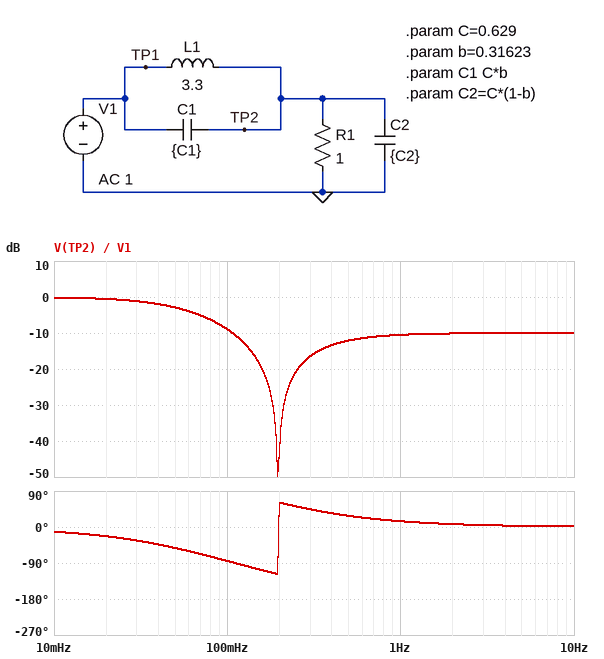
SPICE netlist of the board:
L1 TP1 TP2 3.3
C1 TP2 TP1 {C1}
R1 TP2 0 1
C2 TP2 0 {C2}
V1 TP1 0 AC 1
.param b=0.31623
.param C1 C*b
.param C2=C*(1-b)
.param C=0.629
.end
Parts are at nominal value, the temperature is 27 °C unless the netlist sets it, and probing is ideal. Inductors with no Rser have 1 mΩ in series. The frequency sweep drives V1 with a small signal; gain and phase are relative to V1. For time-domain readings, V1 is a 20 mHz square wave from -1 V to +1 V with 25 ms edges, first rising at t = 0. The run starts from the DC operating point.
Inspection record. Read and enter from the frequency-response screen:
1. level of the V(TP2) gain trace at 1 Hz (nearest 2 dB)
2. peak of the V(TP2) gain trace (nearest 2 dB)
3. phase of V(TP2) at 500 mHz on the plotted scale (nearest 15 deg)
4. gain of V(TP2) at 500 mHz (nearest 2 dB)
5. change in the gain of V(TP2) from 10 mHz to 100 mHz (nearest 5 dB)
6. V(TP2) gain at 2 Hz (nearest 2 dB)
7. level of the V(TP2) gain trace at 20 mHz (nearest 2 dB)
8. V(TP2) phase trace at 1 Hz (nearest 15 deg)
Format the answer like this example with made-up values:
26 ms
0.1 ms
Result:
-10 dB
0 dB
30 deg
-12 dB
-10 dB
-10 dB
0 dB
15 deg
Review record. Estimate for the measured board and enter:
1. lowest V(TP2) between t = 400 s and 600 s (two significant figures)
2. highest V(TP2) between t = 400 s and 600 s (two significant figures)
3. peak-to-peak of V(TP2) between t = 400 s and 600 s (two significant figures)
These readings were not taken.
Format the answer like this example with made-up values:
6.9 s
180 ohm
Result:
-1.0 V
1.0 V
2.0 V
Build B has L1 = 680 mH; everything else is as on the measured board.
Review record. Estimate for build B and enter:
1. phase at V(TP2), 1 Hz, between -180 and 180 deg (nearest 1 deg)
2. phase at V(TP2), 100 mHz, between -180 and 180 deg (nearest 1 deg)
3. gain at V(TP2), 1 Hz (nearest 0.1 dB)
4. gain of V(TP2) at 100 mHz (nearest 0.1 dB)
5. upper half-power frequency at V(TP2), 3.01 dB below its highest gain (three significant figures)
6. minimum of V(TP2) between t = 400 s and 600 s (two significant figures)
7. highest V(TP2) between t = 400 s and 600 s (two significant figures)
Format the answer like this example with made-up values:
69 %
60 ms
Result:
15 deg
-27 deg
-11.6 dB
0.1 dB
232 mHz
-1.2 V
1.2 V
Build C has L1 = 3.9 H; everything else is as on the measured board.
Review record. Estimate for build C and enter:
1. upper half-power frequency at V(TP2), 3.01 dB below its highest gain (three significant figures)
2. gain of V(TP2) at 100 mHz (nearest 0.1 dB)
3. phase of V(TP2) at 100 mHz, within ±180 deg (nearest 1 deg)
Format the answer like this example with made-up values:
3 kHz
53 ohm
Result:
42.9 mHz
-11.0 dB
-89 deg
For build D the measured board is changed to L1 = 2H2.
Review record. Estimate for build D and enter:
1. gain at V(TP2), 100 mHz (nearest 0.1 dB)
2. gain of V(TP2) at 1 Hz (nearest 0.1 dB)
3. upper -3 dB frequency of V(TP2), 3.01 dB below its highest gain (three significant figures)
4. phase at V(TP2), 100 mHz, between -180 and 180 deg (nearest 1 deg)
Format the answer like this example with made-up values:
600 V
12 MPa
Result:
-4.9 dB
-10.6 dB
77.8 mHz
-72 deg
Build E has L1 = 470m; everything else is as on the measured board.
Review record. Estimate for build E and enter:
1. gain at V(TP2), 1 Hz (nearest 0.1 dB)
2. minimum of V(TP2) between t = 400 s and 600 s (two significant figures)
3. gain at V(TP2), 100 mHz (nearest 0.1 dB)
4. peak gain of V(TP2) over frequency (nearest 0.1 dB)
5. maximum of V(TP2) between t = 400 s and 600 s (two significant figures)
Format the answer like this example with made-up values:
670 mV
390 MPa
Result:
-12.3 dB
-1.3 V
0.3 dB
0.6 dB
1.3 V
